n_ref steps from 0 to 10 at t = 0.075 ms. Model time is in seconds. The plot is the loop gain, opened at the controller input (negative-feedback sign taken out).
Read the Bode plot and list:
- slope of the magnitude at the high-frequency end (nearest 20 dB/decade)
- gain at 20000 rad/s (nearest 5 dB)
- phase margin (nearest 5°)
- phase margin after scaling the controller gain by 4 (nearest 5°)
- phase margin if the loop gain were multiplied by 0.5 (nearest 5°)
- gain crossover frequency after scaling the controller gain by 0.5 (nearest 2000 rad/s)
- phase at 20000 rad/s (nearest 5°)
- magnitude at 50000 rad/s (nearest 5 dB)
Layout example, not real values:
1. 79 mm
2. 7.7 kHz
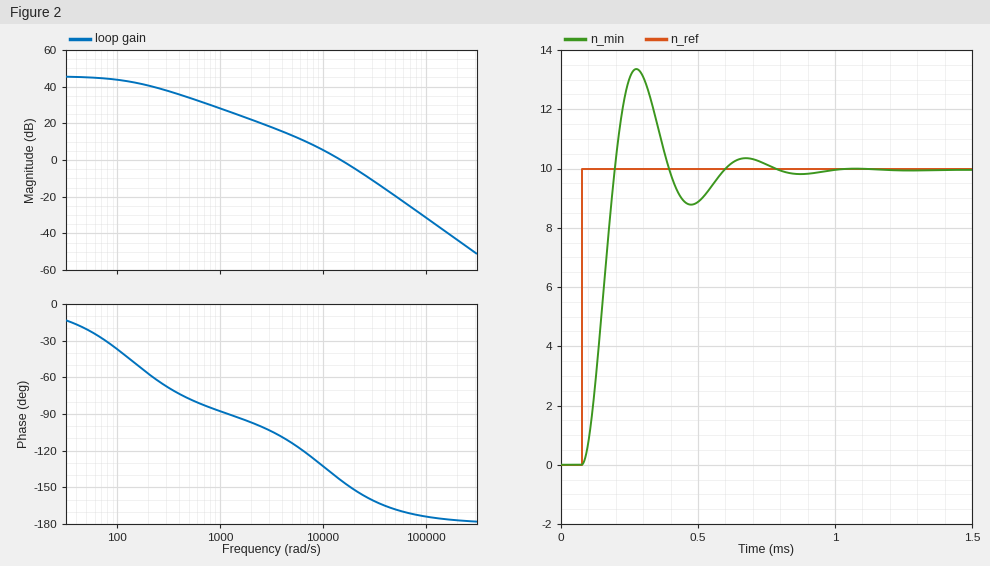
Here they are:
1. -40 dB/decade
2. -5 dB
3. 35°
4. 20°
5. 50°
6. 10000 rad/s
7. -150°
8. -20 dB
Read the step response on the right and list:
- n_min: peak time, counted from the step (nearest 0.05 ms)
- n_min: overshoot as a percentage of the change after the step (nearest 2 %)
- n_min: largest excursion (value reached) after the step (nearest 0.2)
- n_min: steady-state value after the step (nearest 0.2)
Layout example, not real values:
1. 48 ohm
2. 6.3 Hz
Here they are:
1. 0.20 ms
2. 34 %
3. 13.4
4. 10.0
